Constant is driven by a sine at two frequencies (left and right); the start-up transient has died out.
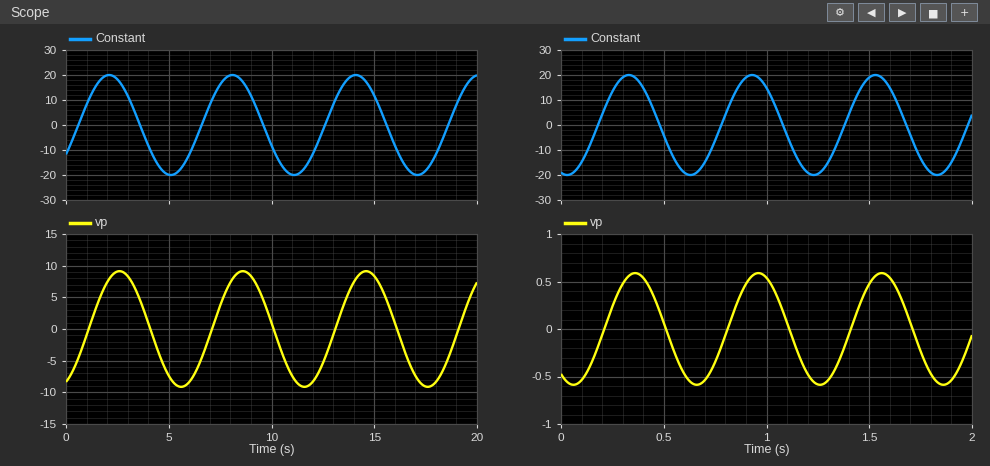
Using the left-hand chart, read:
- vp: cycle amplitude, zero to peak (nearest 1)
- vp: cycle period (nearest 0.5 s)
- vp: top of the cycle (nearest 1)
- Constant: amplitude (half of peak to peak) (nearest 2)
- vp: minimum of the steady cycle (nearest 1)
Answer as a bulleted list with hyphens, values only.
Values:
- 9
- 6.0 s
- 9
- 20
- -9
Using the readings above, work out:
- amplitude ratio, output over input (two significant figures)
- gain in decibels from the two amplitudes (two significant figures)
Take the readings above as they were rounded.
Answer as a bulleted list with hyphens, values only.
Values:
- 0.45
- -6.9 dB
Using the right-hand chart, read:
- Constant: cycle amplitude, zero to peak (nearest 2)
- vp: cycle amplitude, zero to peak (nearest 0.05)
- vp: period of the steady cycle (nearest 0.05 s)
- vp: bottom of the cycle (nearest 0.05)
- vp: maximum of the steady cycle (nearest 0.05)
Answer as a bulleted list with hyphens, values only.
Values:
- 20
- 0.60
- 0.60 s
- -0.60
- 0.60
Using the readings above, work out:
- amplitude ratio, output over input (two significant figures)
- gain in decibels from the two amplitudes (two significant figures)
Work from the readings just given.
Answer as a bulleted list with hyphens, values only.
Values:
- 0.030
- -30 dB
